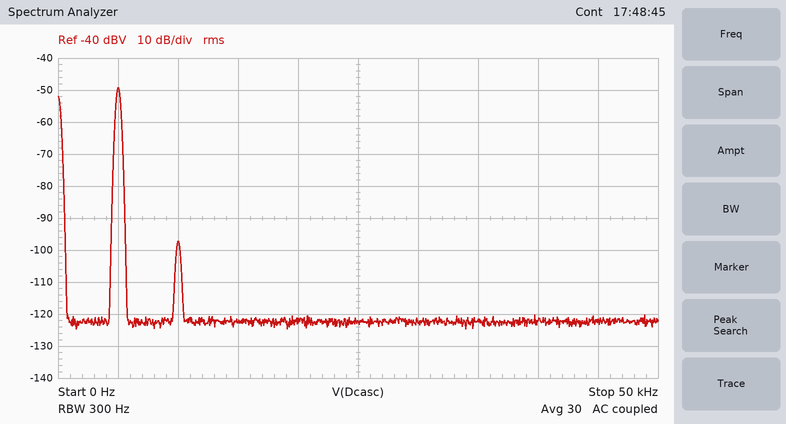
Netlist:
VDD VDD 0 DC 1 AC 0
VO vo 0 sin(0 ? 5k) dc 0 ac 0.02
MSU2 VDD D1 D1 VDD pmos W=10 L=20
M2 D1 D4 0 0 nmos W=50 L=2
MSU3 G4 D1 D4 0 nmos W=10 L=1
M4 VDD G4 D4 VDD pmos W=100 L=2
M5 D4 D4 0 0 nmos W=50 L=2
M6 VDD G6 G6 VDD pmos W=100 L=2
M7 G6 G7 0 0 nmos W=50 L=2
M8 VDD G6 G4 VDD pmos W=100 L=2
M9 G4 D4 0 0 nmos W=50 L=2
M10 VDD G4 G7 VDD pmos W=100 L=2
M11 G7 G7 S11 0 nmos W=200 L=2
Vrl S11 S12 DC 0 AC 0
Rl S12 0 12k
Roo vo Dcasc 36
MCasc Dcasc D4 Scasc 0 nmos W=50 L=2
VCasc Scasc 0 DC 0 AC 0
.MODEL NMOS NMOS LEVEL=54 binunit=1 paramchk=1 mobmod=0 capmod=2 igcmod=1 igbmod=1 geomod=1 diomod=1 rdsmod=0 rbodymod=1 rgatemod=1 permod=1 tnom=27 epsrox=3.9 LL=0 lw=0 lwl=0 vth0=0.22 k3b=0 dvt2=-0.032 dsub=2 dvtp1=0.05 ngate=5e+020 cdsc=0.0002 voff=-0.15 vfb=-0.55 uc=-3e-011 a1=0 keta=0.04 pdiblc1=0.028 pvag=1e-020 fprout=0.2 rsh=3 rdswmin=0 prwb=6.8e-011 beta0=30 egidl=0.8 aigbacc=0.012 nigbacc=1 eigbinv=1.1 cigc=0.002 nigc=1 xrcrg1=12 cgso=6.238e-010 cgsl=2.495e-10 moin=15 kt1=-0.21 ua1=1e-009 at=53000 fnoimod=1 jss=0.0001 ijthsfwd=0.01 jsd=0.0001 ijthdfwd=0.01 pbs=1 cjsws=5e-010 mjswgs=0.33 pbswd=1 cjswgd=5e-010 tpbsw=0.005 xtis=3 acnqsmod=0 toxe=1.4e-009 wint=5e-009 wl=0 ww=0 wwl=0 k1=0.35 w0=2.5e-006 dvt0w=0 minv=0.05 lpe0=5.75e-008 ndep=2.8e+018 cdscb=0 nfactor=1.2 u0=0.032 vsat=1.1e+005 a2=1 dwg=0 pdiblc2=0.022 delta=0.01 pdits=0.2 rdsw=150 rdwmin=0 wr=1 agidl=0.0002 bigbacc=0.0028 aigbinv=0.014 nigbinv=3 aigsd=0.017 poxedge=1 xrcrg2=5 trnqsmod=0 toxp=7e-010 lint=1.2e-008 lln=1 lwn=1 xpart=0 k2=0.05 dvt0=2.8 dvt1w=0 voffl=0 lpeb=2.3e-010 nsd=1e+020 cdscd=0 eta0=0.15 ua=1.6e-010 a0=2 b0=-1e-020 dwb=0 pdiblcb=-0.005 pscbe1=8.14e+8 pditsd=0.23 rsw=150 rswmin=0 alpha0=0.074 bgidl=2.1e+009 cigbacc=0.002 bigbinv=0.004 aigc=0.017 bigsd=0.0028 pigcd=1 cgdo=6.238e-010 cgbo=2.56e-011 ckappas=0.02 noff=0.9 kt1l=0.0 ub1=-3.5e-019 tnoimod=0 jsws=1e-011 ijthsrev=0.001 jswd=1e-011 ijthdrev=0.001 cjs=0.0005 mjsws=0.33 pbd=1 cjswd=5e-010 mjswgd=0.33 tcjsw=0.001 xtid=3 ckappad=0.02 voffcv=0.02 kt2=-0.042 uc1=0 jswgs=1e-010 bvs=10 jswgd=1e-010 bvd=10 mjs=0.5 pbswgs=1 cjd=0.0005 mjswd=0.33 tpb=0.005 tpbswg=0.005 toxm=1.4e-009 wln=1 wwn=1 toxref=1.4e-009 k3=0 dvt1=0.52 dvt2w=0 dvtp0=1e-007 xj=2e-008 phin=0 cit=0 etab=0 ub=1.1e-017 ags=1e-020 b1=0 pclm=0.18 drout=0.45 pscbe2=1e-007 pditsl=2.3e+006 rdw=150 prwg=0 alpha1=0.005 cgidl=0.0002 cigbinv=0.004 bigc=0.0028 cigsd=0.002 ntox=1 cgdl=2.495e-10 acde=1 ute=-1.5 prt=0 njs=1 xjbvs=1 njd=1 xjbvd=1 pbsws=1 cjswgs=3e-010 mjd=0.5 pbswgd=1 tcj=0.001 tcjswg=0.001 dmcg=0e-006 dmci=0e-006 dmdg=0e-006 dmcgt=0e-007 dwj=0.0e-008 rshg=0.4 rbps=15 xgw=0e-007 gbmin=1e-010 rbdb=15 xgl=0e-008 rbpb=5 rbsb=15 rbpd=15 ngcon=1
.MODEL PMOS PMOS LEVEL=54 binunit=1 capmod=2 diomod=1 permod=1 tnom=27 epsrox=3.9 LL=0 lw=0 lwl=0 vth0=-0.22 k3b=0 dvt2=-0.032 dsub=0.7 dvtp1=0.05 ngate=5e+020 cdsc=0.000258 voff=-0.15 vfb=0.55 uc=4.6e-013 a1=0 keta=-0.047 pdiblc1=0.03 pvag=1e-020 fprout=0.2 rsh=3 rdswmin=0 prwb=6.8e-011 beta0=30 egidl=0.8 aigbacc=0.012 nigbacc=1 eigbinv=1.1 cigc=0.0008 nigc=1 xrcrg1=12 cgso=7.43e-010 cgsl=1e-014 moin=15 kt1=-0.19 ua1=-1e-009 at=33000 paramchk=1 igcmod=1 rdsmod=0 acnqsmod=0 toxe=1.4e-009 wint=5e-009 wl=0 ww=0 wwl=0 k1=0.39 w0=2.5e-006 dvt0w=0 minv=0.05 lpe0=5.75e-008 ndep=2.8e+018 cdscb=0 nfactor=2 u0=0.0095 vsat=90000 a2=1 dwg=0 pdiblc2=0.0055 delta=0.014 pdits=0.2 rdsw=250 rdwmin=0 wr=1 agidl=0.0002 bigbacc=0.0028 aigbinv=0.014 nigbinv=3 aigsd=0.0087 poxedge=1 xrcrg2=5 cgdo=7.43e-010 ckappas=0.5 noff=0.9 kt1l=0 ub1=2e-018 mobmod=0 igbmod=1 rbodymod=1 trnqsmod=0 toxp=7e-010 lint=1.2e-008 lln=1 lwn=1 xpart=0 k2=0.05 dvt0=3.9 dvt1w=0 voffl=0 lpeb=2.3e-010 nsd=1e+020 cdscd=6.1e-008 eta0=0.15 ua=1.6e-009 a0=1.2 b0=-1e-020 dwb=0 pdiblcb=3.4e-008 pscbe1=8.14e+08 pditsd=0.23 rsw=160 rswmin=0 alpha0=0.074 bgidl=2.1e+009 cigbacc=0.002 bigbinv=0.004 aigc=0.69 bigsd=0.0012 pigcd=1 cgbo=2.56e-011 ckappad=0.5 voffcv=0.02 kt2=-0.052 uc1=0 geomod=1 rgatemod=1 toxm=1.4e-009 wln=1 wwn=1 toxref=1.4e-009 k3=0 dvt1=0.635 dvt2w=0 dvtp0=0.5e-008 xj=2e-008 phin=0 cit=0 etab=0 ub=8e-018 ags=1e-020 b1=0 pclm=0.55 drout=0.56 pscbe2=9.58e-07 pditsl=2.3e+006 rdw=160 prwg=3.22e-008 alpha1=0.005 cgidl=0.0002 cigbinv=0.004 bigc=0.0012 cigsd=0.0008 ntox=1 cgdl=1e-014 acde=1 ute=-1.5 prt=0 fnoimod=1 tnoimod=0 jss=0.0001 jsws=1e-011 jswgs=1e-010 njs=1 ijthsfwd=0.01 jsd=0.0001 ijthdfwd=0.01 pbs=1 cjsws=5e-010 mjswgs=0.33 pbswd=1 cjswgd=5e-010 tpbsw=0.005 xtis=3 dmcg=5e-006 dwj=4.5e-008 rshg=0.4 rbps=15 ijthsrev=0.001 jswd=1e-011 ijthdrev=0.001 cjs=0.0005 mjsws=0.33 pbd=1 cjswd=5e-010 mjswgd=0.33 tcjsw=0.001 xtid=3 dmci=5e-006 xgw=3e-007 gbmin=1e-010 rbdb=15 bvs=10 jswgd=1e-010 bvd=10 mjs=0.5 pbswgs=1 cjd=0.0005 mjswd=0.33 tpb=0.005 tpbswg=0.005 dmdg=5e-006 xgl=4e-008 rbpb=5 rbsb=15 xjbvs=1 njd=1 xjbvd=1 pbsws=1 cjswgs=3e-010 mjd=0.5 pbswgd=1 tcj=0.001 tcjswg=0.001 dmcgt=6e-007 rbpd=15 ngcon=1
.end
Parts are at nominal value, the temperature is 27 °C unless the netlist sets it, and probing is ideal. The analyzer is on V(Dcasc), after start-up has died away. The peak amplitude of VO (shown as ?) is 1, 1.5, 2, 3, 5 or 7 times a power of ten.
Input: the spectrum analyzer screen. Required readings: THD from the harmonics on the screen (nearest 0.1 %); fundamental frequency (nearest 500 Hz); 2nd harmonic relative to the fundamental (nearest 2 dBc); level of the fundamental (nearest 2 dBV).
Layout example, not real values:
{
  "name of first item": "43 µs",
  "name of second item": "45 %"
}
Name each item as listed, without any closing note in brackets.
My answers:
{
  "THD from the harmonics on the screen": "0.4 %",
  "fundamental frequency": "5.0 kHz",
  "2nd harmonic relative to the fundamental": "-48 dBc",
  "level of the fundamental": "-50 dBV"
}
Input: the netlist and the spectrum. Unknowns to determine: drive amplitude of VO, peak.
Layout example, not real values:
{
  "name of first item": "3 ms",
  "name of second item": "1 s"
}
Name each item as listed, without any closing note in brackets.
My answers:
{
  "drive amplitude of VO, peak": "15 mV"
}
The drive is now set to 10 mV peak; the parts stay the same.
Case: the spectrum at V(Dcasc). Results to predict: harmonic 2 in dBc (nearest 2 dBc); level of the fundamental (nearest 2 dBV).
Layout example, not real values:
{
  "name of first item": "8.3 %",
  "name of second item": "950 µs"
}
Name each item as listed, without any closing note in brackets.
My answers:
{
  "harmonic 2 in dBc": "-52 dBc",
  "level of the fundamental": "-52 dBV"
}
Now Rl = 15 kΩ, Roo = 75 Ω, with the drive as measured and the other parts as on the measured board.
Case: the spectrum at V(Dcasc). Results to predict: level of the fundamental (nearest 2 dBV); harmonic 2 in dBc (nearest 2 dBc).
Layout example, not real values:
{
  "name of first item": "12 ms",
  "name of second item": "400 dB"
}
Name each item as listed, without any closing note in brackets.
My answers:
{
  "level of the fundamental": "-58 dBV",
  "harmonic 2 in dBc": "-56 dBc"
}
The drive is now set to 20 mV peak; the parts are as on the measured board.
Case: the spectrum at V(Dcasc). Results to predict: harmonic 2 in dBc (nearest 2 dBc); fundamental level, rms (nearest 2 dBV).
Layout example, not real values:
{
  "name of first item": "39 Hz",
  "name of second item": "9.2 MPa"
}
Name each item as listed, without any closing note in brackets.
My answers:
{
  "harmonic 2 in dBc": "-46 dBc",
  "fundamental level, rms": "-46 dBV"
}
